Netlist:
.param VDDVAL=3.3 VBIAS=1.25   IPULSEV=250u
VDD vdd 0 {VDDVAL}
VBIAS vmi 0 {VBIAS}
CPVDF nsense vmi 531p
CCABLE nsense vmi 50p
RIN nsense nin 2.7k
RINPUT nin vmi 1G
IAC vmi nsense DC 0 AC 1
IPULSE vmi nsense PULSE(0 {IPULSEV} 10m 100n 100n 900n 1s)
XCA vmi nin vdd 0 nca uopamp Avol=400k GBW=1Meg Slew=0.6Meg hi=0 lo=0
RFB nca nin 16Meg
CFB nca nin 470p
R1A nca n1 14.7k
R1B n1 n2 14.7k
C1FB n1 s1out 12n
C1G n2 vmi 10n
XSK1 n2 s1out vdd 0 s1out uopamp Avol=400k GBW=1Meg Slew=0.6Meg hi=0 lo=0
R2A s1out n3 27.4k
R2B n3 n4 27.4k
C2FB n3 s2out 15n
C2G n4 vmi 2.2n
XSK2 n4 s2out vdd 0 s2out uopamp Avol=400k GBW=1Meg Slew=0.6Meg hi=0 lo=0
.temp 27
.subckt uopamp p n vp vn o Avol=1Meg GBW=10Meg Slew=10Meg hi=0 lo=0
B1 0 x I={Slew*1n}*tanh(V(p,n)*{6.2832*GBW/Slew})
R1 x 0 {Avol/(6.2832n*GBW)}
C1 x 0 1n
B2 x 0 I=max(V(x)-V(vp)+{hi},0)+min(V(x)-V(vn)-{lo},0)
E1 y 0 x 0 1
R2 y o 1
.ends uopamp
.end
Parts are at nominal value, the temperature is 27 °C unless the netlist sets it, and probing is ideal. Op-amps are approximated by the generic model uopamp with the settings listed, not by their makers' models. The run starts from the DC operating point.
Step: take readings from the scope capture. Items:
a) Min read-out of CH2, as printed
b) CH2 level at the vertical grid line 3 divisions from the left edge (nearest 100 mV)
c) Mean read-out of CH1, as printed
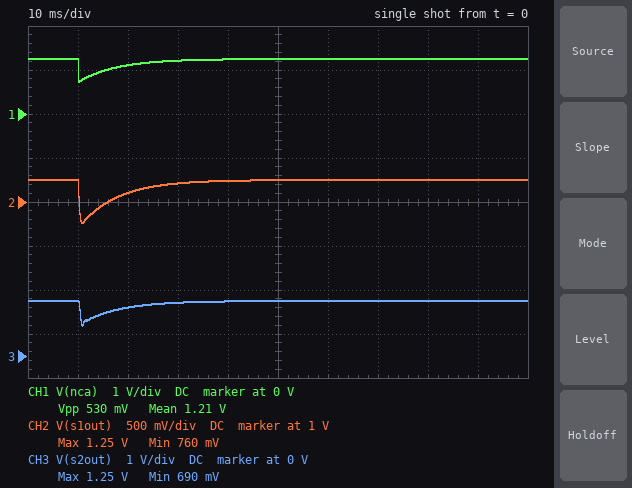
760 mV
1.2 V
1.21 V
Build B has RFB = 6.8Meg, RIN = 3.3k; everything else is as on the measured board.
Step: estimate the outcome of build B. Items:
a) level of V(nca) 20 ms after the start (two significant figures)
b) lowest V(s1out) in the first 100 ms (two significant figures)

1.2 V
800 mV
